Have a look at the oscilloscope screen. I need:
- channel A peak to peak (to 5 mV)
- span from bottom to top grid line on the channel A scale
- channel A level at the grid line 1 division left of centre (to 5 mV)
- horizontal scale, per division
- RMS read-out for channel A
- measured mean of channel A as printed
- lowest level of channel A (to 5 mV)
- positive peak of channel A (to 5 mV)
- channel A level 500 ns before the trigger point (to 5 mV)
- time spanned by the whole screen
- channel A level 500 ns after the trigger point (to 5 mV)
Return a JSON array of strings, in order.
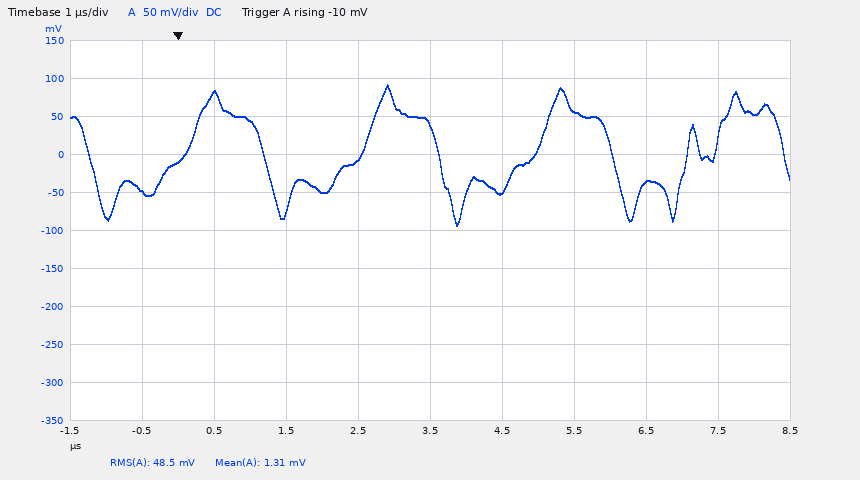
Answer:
["185 mV", "500 mV", "-5 mV", "1 µs", "48.5 mV", "1.31 mV", "-95 mV", "90 mV", "-50 mV", "10 µs", "80 mV"]
